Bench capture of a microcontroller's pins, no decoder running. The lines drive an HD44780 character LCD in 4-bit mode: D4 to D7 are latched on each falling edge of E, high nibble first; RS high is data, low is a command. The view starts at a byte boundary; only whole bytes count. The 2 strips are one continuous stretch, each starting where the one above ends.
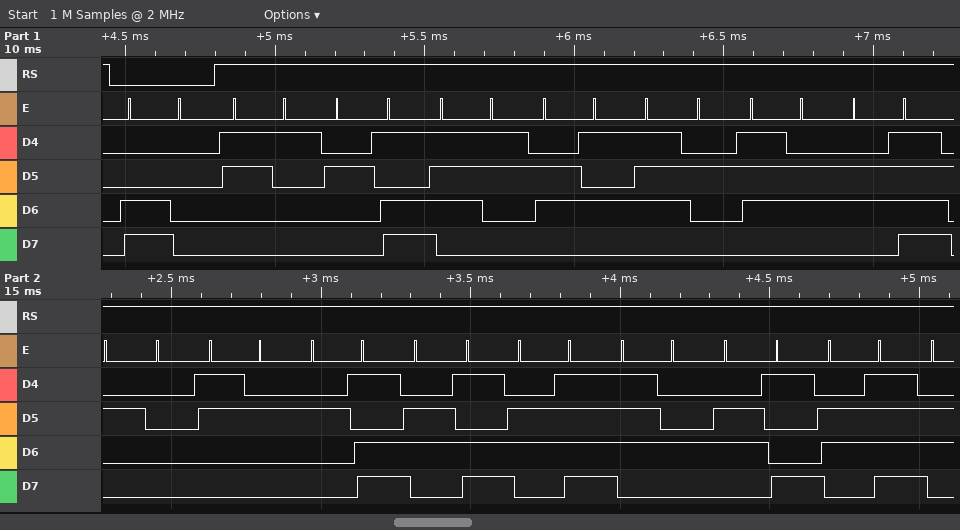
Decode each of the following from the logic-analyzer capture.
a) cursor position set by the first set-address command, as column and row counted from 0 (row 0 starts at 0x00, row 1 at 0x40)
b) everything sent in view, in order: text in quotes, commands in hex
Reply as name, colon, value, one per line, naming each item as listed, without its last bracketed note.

cursor position set by the first set-address command, as column and row counted from 0: column 0, row 1
everything sent in view, in order: text in quotes, commands in hex: 0xC0 "1-servo 2-motio"
